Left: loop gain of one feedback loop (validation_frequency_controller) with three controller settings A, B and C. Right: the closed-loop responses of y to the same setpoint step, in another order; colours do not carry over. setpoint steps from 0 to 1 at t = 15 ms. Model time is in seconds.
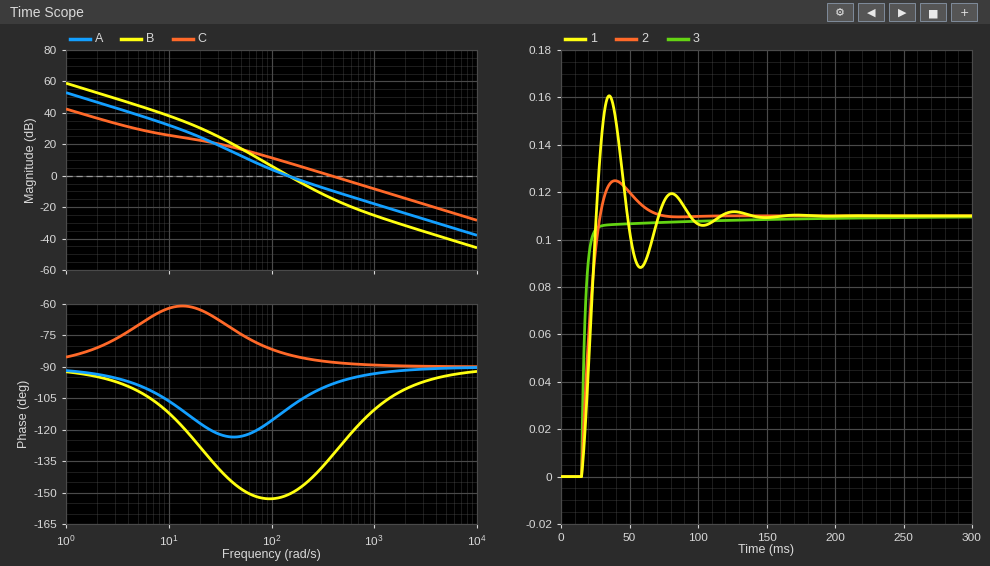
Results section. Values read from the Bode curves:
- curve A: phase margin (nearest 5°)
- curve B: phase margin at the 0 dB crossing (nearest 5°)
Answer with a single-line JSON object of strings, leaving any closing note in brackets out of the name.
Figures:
{"curve A: phase margin": "70°", "curve B: phase margin at the 0 dB crossing": "30°"}
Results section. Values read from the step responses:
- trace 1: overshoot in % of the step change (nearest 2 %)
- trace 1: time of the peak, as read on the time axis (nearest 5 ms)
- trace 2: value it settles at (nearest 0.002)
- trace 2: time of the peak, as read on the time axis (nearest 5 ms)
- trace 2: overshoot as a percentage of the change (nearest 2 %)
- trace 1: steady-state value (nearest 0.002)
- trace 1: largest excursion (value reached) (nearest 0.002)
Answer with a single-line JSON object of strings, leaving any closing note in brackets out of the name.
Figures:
{"trace 1: overshoot in % of the step change": "46 %", "trace 1: time of the peak, as read on the time axis": "35 ms", "trace 2: value it settles at": "0.110", "trace 2: time of the peak, as read on the time axis": "40 ms", "trace 2: overshoot as a percentage of the change": "14 %", "trace 1: steady-state value": "0.110", "trace 1: largest excursion (value reached)": "0.160"}
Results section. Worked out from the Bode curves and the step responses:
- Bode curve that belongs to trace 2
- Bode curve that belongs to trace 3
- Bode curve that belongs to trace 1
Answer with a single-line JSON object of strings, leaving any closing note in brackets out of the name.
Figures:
{"Bode curve that belongs to trace 2": "A", "Bode curve that belongs to trace 3": "C", "Bode curve that belongs to trace 1": "B"}
